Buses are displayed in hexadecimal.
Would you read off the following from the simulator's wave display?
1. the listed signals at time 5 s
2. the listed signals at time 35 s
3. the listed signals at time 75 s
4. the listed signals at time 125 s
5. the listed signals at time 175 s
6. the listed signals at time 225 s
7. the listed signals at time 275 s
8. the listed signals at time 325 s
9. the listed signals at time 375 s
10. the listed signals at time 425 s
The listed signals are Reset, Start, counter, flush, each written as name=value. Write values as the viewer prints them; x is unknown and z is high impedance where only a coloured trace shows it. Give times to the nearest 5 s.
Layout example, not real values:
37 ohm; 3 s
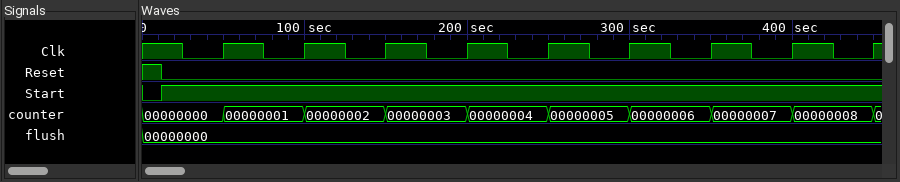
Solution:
Reset=1, Start=0, counter=00000000, flush=00000000; Reset=0, Start=1, counter=00000000, flush=00000000; Reset=0, Start=1, counter=00000001, flush=00000000; Reset=0, Start=1, counter=00000002, flush=00000000; Reset=0, Start=1, counter=00000003, flush=00000000; Reset=0, Start=1, counter=00000004, flush=00000000; Reset=0, Start=1, counter=00000005, flush=00000000; Reset=0, Start=1, counter=00000006, flush=00000000; Reset=0, Start=1, counter=00000007, flush=00000000; Reset=0, Start=1, counter=00000008, flush=00000000
